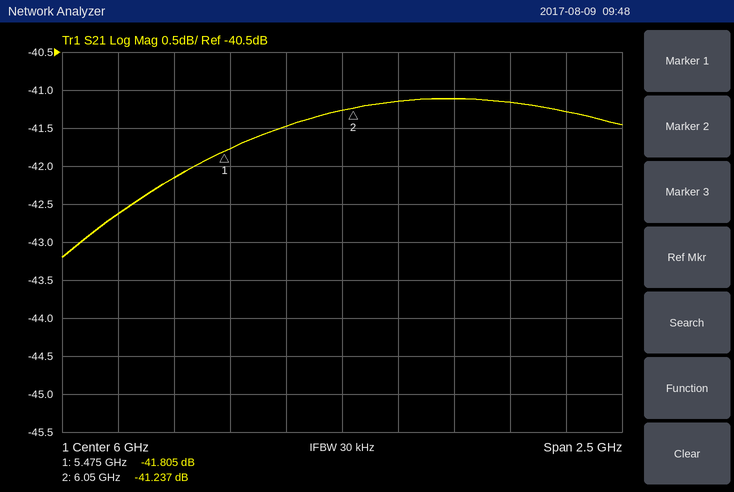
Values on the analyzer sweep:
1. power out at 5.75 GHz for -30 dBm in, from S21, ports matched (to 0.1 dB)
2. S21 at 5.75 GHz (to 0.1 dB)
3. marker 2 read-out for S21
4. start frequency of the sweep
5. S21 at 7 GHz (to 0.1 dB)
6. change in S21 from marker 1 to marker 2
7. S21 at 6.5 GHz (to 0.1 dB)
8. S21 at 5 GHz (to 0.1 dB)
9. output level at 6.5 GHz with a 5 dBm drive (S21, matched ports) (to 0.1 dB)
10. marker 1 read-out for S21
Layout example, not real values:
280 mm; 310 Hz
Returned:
-71.5 dBm; -41.5 dB; -41.237 dB; 4.75 GHz; -41.3 dB; 0.568 dB; -41.1 dB; -42.6 dB; -36.1 dBm; -41.805 dB
